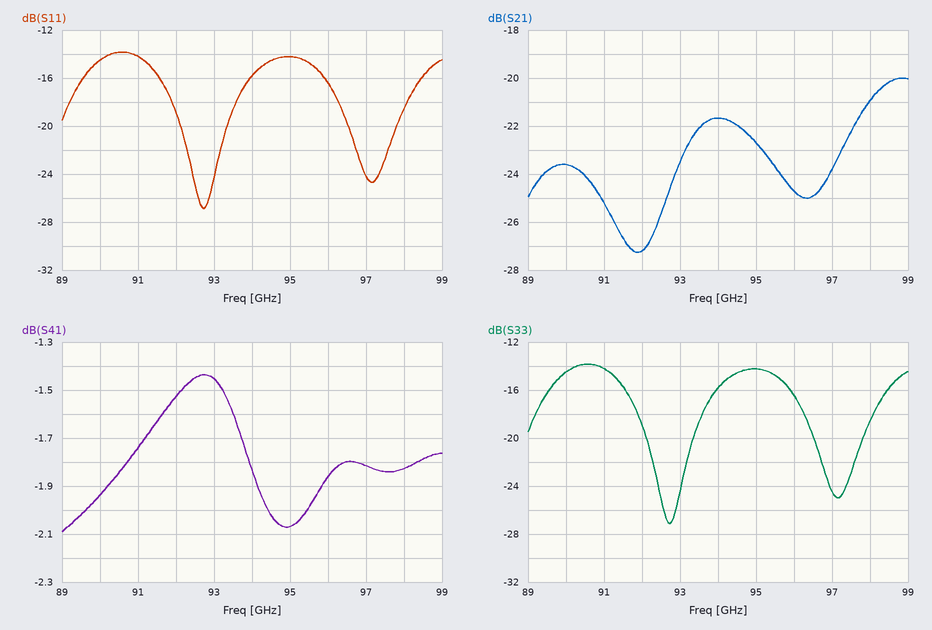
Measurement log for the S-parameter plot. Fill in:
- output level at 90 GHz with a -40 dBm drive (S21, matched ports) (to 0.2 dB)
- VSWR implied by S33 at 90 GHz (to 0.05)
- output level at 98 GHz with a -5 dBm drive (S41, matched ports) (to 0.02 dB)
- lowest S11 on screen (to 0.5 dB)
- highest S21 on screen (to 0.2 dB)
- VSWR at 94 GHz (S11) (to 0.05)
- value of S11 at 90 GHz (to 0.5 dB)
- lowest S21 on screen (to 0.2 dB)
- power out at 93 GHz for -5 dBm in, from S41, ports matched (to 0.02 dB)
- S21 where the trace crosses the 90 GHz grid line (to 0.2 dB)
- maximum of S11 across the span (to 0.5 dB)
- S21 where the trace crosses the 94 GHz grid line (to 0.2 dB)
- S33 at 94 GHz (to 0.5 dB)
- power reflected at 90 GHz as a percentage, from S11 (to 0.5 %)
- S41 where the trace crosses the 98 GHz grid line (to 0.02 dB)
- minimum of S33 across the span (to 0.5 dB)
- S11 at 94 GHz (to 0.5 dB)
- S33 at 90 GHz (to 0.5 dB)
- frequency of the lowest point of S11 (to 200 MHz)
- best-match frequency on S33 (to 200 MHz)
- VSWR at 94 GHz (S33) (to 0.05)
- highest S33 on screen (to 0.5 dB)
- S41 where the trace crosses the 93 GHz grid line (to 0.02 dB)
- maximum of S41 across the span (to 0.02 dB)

-63.6 dBm
1.45
-6.82 dBm
-27.0 dB
-20.0 dB
1.40
-14.5 dB
-27.2 dB
-6.46 dBm
-23.6 dB
-14.0 dB
-21.6 dB
-16.0 dB
3.5 %
-1.82 dB
-27.0 dB
-16.0 dB
-14.5 dB
92.8 GHz
92.8 GHz
1.40
-14.0 dB
-1.46 dB
-1.44 dB
